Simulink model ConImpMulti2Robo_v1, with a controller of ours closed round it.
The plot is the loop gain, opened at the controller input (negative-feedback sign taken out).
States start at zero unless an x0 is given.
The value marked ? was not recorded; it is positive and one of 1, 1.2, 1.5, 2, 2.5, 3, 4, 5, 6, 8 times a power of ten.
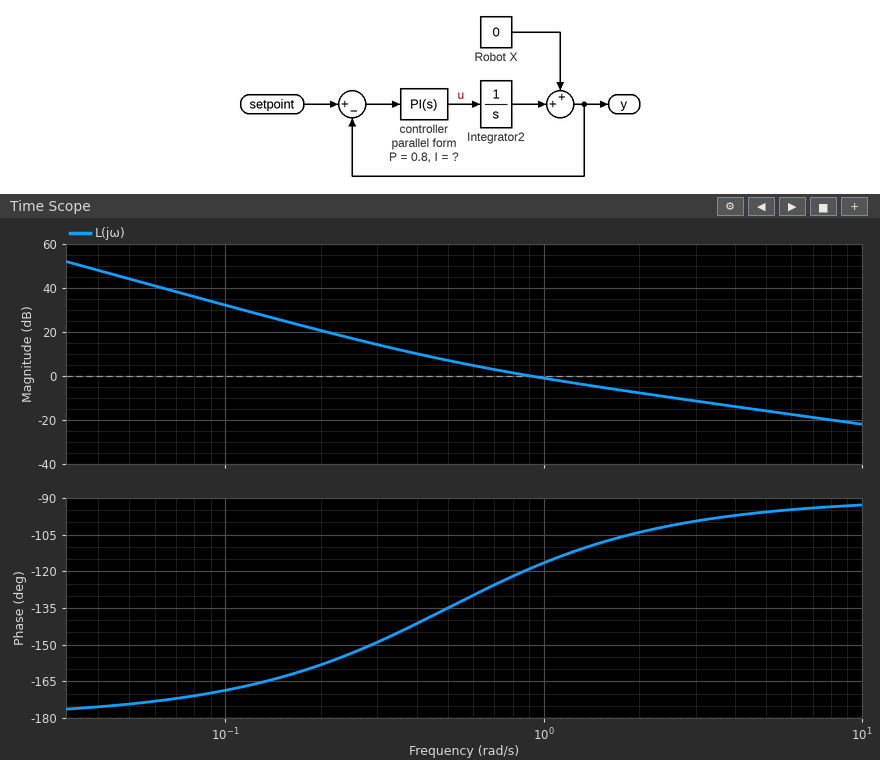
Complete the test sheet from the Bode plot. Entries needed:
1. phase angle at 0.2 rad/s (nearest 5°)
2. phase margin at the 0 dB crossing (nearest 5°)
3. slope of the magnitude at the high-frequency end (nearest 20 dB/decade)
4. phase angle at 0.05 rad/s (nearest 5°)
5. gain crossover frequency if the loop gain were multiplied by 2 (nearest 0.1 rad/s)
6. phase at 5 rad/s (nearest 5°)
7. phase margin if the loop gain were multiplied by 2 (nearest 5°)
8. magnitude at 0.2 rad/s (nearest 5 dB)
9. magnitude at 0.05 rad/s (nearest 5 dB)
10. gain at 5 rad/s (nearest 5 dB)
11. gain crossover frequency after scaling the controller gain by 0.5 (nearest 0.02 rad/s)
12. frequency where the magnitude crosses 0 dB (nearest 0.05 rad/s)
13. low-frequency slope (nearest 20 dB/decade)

-160°
60°
-20 dB/decade
-175°
1.7 rad/s
-95°
75°
20 dB
45 dB
-15 dB
0.54 rad/s
0.90 rad/s
-40 dB/decade
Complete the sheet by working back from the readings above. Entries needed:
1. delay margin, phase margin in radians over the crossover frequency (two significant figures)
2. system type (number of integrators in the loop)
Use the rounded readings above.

1.2 s
2
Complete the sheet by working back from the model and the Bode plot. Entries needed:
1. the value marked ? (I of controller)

0.4
